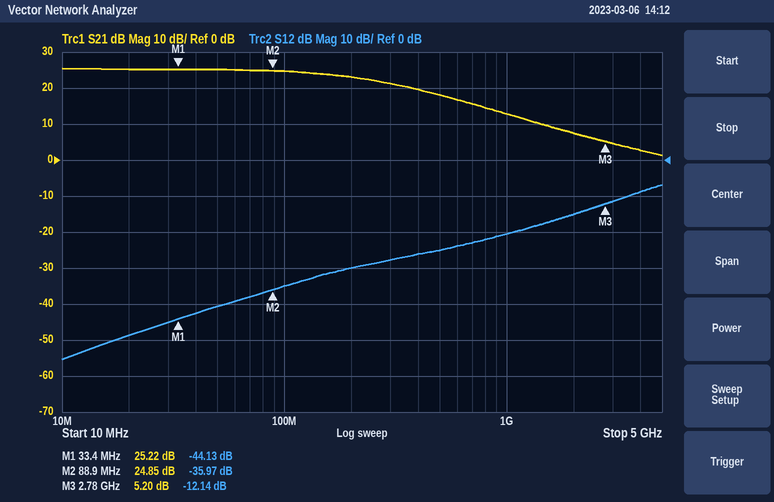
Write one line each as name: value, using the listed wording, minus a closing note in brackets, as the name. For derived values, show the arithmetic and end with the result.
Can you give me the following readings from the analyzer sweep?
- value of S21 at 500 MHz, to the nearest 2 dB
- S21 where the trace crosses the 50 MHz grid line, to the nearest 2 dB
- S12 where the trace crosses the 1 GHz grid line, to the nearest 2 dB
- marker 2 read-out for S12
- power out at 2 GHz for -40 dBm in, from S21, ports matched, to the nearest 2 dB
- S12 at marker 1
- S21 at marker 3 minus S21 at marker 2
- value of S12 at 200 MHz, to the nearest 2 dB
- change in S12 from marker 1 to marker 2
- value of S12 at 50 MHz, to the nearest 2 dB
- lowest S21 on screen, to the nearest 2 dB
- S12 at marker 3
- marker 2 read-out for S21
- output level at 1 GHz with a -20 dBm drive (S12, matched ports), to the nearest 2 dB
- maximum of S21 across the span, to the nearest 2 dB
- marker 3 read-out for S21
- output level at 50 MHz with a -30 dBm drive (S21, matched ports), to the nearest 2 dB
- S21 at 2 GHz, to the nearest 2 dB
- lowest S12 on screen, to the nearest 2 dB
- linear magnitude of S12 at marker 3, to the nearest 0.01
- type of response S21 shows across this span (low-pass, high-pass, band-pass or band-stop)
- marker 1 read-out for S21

value of S21 at 500 MHz, to the nearest 2 dB: 18 dB
S21 where the trace crosses the 50 MHz grid line, to the nearest 2 dB: 26 dB
S12 where the trace crosses the 1 GHz grid line, to the nearest 2 dB: -20 dB
marker 2 read-out for S12: -35.97 dB
power out at 2 GHz for -40 dBm in, from S21, ports matched, to the nearest 2 dB: -40 dBm + (8 dB) = -32 dBm
S12 at marker 1: -44.13 dB
S21 at marker 3 minus S21 at marker 2: 5.2 − (24.85) = -19.65 dB
value of S12 at 200 MHz, to the nearest 2 dB: -30 dB
change in S12 from marker 1 to marker 2: -35.97 − (-44.13) = 8.16 dB
value of S12 at 50 MHz, to the nearest 2 dB: -40 dB
lowest S21 on screen, to the nearest 2 dB: 2 dB
S12 at marker 3: -12.14 dB
marker 2 read-out for S21: 24.85 dB
output level at 1 GHz with a -20 dBm drive (S12, matched ports), to the nearest 2 dB: -20 dBm + (-20 dB) = -40 dBm
maximum of S21 across the span, to the nearest 2 dB: 26 dB
marker 3 read-out for S21: 5.20 dB
output level at 50 MHz with a -30 dBm drive (S21, matched ports), to the nearest 2 dB: -30 dBm + (26 dB) = -4 dBm
S21 at 2 GHz, to the nearest 2 dB: 8 dB
lowest S12 on screen, to the nearest 2 dB: -56 dB
linear magnitude of S12 at marker 3, to the nearest 0.01: 10^(-12.14/20) ≈ 0.25
type of response S21 shows across this span: low-pass
marker 1 read-out for S21: 25.22 dB
